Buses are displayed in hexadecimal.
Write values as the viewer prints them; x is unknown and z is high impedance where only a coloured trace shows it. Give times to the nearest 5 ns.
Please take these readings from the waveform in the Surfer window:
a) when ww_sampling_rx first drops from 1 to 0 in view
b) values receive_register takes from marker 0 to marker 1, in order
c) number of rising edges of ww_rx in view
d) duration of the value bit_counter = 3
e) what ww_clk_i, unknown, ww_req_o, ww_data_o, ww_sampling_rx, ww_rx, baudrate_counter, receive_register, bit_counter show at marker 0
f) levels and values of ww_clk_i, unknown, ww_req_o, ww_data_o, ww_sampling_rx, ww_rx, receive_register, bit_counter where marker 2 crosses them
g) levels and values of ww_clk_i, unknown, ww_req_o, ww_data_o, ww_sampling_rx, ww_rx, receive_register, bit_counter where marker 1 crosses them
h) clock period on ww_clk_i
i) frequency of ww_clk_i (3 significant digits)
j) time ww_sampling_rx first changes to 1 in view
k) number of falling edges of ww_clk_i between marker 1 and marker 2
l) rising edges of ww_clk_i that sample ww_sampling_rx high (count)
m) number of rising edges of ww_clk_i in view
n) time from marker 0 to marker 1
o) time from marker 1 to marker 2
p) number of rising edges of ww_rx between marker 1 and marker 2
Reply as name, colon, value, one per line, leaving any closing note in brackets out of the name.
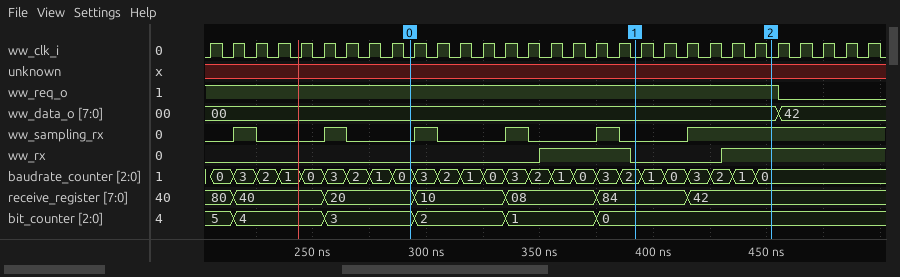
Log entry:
when ww_sampling_rx first drops from 1 to 0 in view: 225 ns
values receive_register takes from marker 0 to marker 1, in order: 20, 10, 08, 84
number of rising edges of ww_rx in view: 2
duration of the value bit_counter = 3: 40 ns
what ww_clk_i, unknown, ww_req_o, ww_data_o, ww_sampling_rx, ww_rx, baudrate_counter, receive_register, bit_counter show at marker 0: ww_clk_i=0, unknown=x, ww_req_o=1, ww_data_o=00, ww_sampling_rx=0, ww_rx=0, baudrate_counter=0, receive_register=20, bit_counter=3
levels and values of ww_clk_i, unknown, ww_req_o, ww_data_o, ww_sampling_rx, ww_rx, receive_register, bit_counter where marker 2 crosses them: ww_clk_i=0, unknown=x, ww_req_o=1, ww_data_o=00, ww_sampling_rx=1, ww_rx=1, receive_register=42, bit_counter=0
levels and values of ww_clk_i, unknown, ww_req_o, ww_data_o, ww_sampling_rx, ww_rx, receive_register, bit_counter where marker 1 crosses them: ww_clk_i=0, unknown=x, ww_req_o=1, ww_data_o=00, ww_sampling_rx=0, ww_rx=0, receive_register=84, bit_counter=0
clock period on ww_clk_i: 10 ns
frequency of ww_clk_i: 100 MHz
time ww_sampling_rx first changes to 1 in view: 215 ns
number of falling edges of ww_clk_i between marker 1 and marker 2: 6
rising edges of ww_clk_i that sample ww_sampling_rx high: 13
number of rising edges of ww_clk_i in view: 30
time from marker 0 to marker 1: 100 ns
time from marker 1 to marker 2: 60 ns
number of rising edges of ww_rx between marker 1 and marker 2: 1
